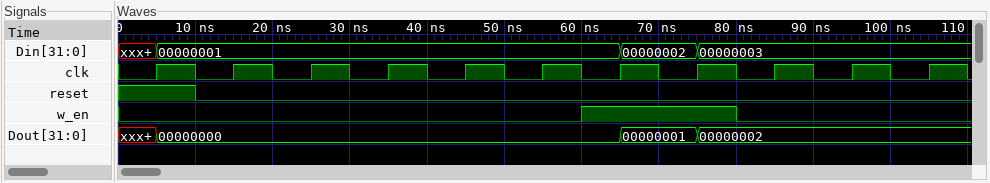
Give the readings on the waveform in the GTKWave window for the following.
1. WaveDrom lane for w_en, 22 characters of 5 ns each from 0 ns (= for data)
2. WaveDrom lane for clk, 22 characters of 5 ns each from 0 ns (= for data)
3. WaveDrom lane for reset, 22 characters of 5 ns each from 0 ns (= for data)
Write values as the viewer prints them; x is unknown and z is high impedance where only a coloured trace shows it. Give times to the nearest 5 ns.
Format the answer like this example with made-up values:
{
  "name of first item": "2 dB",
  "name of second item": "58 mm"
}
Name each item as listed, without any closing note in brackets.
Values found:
{
  "WaveDrom lane for w_en, 22 characters of 5 ns each from 0 ns": "{name: 'w_en', wave: '0...........1...0.....'}",
  "WaveDrom lane for clk, 22 characters of 5 ns each from 0 ns": "{name: 'clk', wave: '0101010101010101010101'}",
  "WaveDrom lane for reset, 22 characters of 5 ns each from 0 ns": "{name: 'reset', wave: '1.0...................'}"
}
